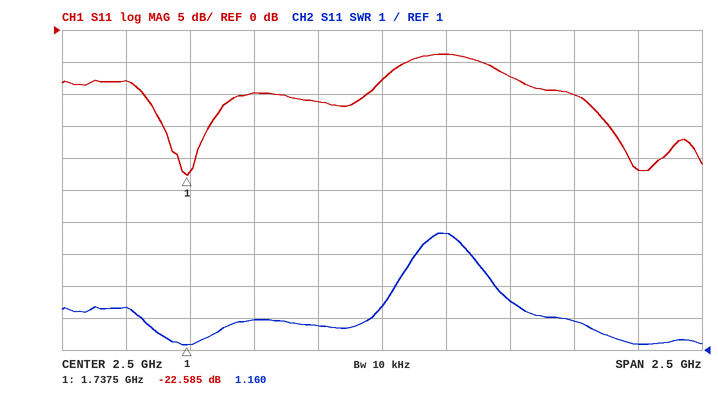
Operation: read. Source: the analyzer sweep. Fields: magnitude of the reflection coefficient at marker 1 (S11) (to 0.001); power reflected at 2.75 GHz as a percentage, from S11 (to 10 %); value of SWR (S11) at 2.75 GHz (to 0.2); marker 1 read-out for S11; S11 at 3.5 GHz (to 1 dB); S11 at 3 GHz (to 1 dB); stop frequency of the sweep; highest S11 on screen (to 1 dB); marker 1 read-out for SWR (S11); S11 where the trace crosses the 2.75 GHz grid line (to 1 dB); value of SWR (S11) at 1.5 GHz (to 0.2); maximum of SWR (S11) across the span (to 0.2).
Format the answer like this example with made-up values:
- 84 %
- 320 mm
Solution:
- 0.074
- 40 %
- 4.6
- -22.585 dB
- -22 dB
- -7 dB
- 3.75 GHz
- -4 dB
- 1.160
- -4 dB
- 2.4
- 4.6
